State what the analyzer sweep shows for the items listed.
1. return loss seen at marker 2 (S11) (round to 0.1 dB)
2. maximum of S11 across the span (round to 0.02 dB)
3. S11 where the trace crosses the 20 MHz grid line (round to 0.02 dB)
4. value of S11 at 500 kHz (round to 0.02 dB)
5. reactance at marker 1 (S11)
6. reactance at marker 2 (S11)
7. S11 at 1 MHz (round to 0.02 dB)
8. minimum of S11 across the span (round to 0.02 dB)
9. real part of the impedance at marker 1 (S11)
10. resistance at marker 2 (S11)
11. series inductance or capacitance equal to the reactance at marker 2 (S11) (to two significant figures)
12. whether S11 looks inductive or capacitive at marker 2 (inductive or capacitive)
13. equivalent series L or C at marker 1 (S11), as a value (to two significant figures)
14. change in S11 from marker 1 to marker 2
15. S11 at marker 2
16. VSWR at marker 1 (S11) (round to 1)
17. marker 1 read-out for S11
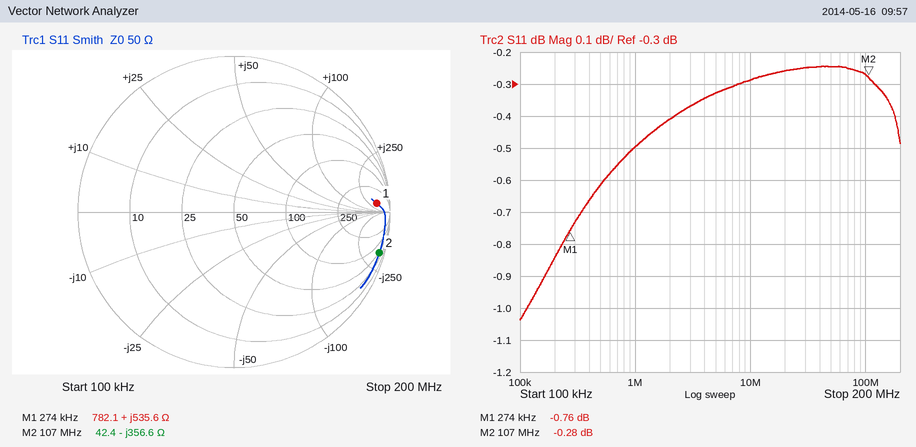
0.3 dB
-0.24 dB
-0.26 dB
-0.62 dB
+535.6 Ω
-356.6 Ω
-0.50 dB
-1.04 dB
782.1 Ω
42.4 Ω
4.2 pF
capacitive
310 µH
0.48 dB
-0.28 dB
23
-0.76 dB
